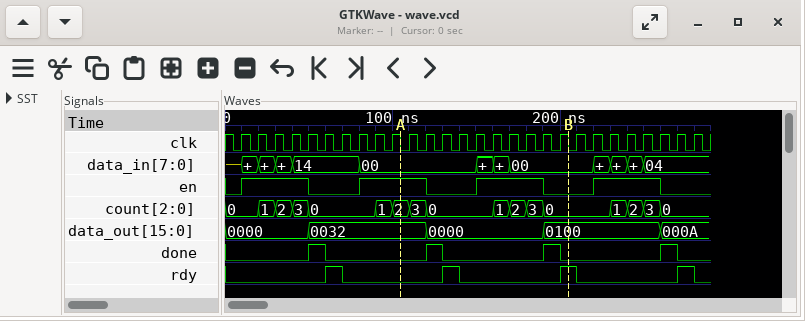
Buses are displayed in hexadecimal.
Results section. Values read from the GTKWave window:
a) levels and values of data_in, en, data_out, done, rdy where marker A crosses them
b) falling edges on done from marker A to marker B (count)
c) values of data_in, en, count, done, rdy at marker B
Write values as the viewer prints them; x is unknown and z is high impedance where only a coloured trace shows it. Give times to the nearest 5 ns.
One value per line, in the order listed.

data_in=00, en=1, data_out=0032, done=0, rdy=0
2
data_in=00, en=0, count=0, done=0, rdy=1
